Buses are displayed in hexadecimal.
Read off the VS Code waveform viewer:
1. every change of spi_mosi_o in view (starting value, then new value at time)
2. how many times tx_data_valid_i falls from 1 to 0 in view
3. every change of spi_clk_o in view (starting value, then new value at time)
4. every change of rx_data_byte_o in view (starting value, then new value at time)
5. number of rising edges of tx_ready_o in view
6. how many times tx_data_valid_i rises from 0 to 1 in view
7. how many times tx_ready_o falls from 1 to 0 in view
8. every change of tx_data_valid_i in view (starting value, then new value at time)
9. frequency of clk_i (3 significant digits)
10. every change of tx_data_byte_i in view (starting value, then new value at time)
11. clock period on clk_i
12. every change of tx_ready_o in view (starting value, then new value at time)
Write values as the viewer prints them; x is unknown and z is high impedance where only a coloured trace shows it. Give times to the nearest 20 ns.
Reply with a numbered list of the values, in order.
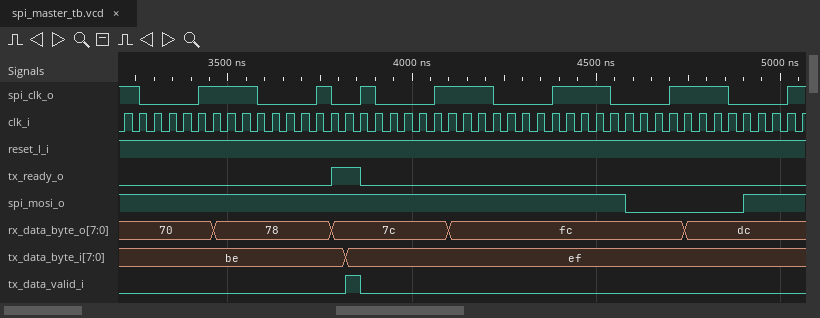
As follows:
1. 1, 0 at 4580 ns, 1 at 4900 ns
2. 1
3. 1, 0 at 3260 ns, 1 at 3420 ns, 0 at 3580 ns, 1 at 3740 ns, 0 at 3780 ns, 1 at 3860 ns, 0 at 3900 ns, 1 at 4060 ns, 0 at 4220 ns, 1 at 4380 ns, 0 at 4540 ns, 1 at 4700 ns, 0 at 4860 ns, 1 at 5020 ns
4. 70, 78 at 3460 ns, 7c at 3780 ns, fc at 4100 ns, dc at 4740 ns
5. 1
6. 1
7. 1
8. 0, 1 at 3820 ns, 0 at 3860 ns
9. 25.0 MHz
10. be, ef at 3820 ns
11. 40 ns
12. 0, 1 at 3780 ns, 0 at 3860 ns
